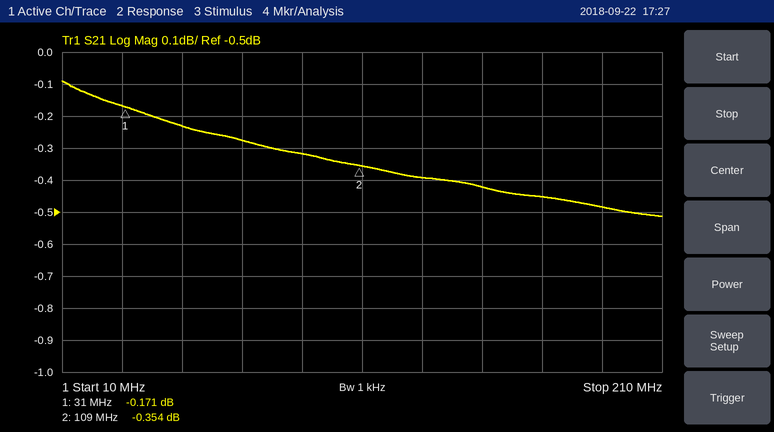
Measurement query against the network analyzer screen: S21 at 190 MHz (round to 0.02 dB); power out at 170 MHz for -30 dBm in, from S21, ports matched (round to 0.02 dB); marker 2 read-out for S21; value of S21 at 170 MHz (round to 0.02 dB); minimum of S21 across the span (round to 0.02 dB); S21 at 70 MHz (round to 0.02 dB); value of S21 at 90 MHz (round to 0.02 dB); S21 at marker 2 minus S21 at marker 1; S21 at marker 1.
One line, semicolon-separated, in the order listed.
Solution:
-0.48 dB; -30.46 dBm; -0.354 dB; -0.46 dB; -0.52 dB; -0.28 dB; -0.32 dB; -0.183 dB; -0.171 dB
